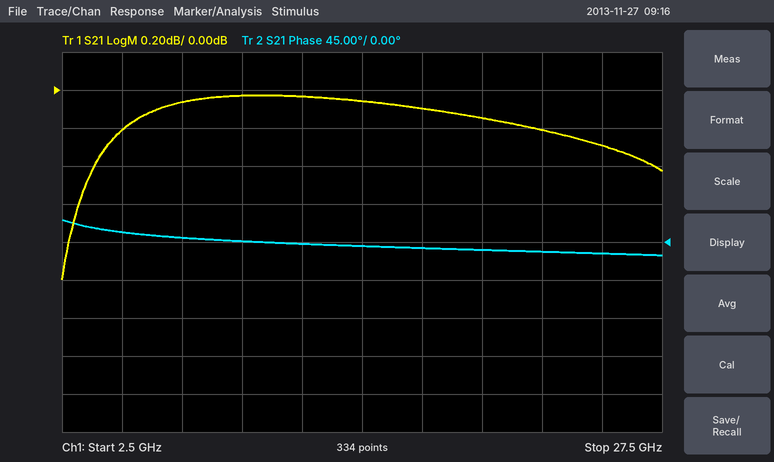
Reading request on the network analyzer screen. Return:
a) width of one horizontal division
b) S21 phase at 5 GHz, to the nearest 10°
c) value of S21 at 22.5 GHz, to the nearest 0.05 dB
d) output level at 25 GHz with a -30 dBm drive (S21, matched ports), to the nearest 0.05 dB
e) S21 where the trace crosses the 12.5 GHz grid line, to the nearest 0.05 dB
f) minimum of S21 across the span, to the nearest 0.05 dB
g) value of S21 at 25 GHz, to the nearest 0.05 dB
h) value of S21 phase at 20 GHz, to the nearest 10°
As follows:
2.5 GHz
10°
-0.20 dB
-30.30 dBm
-0.05 dB
-1.00 dB
-0.30 dB
-10°
